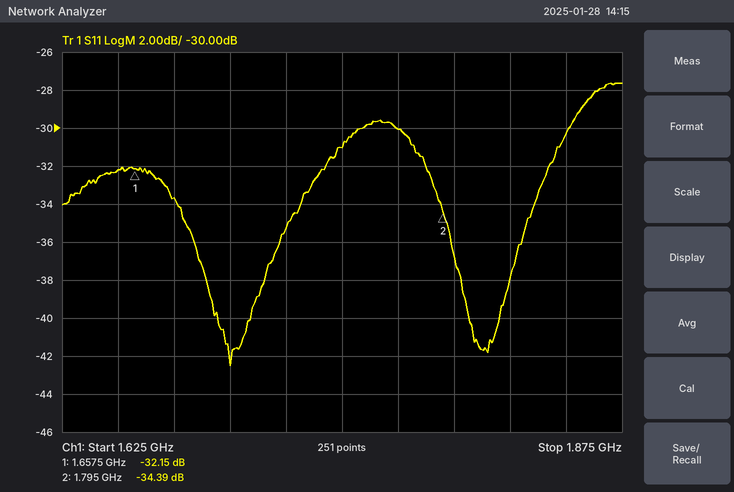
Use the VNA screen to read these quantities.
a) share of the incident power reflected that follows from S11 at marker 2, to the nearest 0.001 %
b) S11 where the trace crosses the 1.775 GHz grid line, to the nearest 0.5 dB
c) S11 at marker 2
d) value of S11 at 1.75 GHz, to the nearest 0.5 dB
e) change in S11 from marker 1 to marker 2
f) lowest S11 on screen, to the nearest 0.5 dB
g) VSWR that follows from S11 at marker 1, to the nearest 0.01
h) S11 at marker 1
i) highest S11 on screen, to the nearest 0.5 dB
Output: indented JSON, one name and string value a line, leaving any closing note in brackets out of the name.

{
  "share of the incident power reflected that follows from S11 at marker 2, to the nearest 0.001 %": "0.036 %",
  "S11 where the trace crosses the 1.775 GHz grid line, to the nearest 0.5 dB": "-30.0 dB",
  "S11 at marker 2": "-34.39 dB",
  "value of S11 at 1.75 GHz, to the nearest 0.5 dB": "-31.0 dB",
  "change in S11 from marker 1 to marker 2": "-2.24 dB",
  "lowest S11 on screen, to the nearest 0.5 dB": "-42.5 dB",
  "VSWR that follows from S11 at marker 1, to the nearest 0.01": "1.05",
  "S11 at marker 1": "-32.15 dB",
  "highest S11 on screen, to the nearest 0.5 dB": "-27.5 dB"
}
